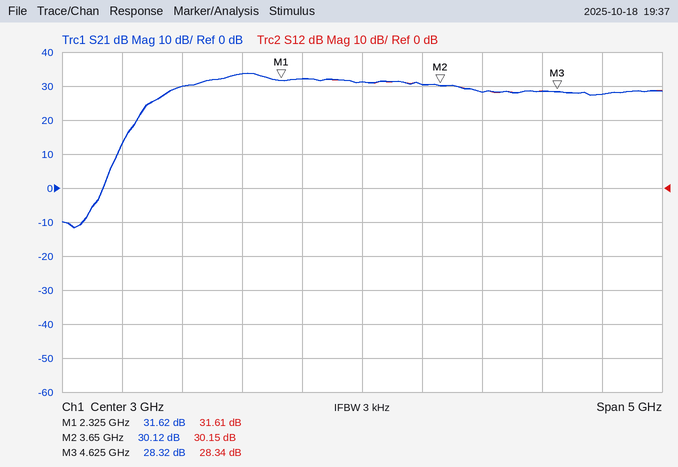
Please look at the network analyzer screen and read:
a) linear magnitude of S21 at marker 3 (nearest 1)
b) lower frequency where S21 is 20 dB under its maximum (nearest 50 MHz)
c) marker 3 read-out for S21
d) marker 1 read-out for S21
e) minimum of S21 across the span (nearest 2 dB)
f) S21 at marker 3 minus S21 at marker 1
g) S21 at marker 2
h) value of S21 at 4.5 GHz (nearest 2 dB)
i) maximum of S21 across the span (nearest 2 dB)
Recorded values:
26
1.00 GHz
28.32 dB
31.62 dB
-12 dB
-3.30 dB
30.12 dB
28 dB
34 dB
